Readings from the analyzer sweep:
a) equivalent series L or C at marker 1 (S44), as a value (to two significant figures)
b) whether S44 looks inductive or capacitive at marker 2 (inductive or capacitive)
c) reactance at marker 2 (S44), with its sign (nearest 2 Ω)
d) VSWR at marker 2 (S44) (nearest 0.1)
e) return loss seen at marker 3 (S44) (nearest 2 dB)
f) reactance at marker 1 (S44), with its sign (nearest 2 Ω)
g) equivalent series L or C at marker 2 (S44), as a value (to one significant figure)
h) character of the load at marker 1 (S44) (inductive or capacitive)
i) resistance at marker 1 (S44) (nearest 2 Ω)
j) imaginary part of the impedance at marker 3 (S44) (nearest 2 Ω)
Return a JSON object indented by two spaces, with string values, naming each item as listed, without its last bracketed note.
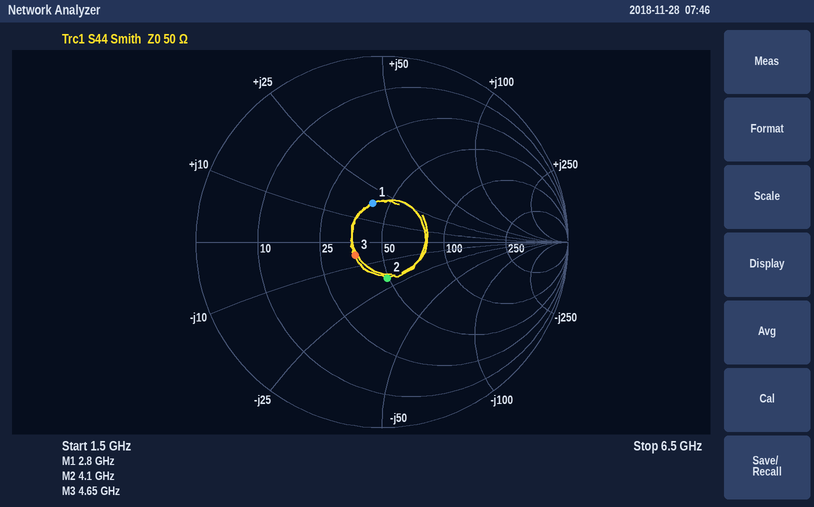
{
  "equivalent series L or C at marker 1 (S44), as a value": "1.0 nH",
  "whether S44 looks inductive or capacitive at marker 2": "capacitive",
  "reactance at marker 2 (S44), with its sign": "-20 Ω",
  "VSWR at marker 2 (S44)": "1.5",
  "return loss seen at marker 3 (S44)": "16 dB",
  "reactance at marker 1 (S44), with its sign": "+18 Ω",
  "equivalent series L or C at marker 2 (S44), as a value": "2 pF",
  "character of the load at marker 1 (S44)": "inductive",
  "resistance at marker 1 (S44)": "42 Ω",
  "imaginary part of the impedance at marker 3 (S44)": "-6 Ω"
}
